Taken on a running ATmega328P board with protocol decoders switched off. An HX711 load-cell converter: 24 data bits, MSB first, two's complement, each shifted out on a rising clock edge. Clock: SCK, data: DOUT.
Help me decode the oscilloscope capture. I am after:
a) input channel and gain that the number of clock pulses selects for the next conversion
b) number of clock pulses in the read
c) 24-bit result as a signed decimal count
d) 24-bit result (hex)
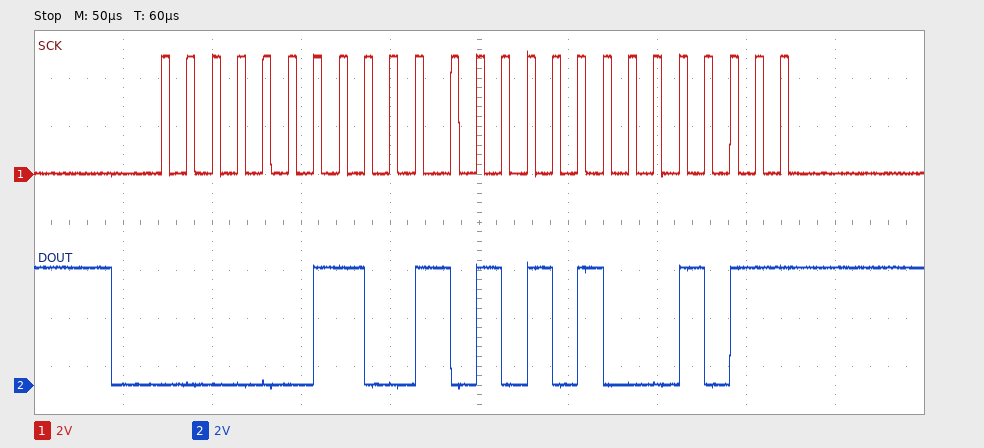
channel A, gain 128
25
207499
0x032A8B
